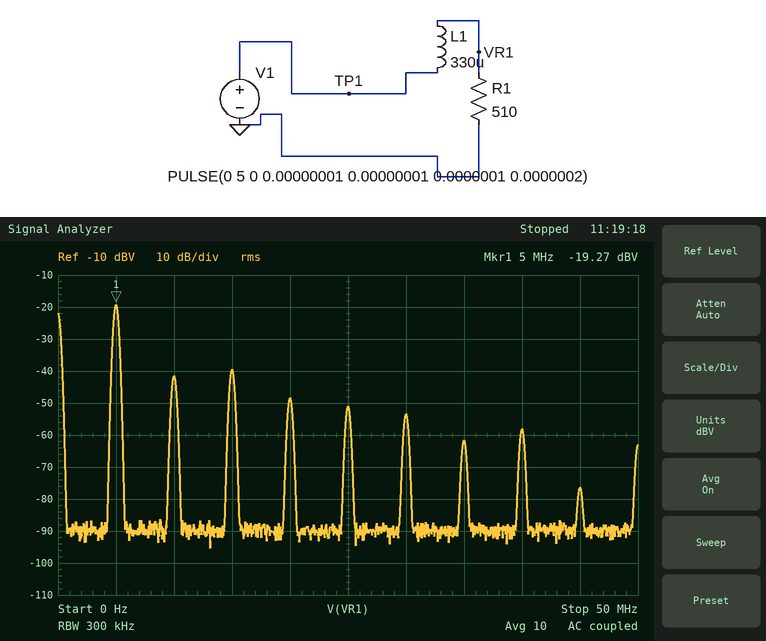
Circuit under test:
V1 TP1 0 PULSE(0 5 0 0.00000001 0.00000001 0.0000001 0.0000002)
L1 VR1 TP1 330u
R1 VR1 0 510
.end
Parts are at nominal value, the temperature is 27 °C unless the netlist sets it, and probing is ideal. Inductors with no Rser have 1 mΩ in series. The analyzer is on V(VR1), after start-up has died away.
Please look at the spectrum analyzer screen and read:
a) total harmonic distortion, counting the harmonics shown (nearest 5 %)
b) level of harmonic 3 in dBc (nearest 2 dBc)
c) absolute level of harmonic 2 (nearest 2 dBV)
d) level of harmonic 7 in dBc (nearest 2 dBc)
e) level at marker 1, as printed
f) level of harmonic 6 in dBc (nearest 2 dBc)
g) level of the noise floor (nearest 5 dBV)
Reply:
15 %
-20 dBc
-42 dBV
-42 dBc
-19.27 dBV
-34 dBc
-90 dBV
